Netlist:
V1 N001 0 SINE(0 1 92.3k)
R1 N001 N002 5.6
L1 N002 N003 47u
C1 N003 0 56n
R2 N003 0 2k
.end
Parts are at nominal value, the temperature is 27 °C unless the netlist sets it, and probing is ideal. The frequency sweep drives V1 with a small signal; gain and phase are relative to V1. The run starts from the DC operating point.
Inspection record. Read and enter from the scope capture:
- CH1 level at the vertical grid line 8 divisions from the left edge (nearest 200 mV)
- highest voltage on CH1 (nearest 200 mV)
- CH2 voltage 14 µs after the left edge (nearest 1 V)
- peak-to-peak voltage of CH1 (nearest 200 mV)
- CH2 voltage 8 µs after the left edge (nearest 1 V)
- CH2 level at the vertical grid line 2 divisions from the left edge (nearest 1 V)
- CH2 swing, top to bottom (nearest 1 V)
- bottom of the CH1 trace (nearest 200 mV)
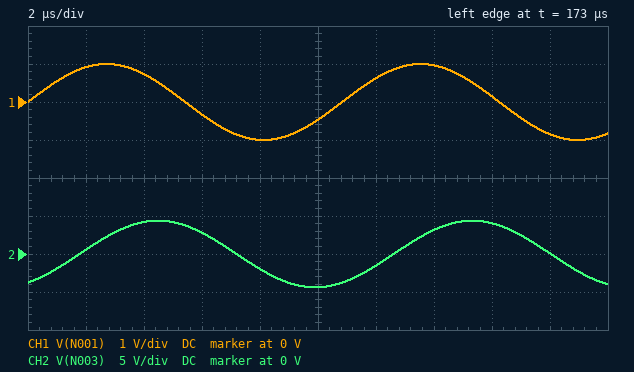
200 mV
1.0 V
3 V
2.0 V
-2 V
4 V
9 V
-1.0 V
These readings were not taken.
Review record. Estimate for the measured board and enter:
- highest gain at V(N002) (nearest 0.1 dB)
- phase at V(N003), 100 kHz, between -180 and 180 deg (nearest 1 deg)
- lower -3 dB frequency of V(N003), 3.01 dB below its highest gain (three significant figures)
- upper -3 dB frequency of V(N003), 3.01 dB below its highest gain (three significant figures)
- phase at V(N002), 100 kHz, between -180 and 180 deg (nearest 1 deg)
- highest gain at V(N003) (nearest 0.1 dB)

0 dB
-100 deg
86.3 kHz
107 kHz
60 deg
13.7 dB
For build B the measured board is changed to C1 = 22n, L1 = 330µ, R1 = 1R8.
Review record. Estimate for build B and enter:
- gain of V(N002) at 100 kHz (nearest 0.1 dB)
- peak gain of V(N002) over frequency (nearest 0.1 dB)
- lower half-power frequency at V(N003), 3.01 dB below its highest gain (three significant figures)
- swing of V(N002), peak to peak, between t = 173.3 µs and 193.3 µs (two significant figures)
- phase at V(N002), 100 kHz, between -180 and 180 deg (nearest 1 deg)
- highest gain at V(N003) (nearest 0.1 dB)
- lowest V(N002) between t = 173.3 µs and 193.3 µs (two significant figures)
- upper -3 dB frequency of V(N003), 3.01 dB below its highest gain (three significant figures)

0 dB
0 dB
56.7 kHz
2.0 V
1 deg
22.4 dB
-1.0 V
61.2 kHz
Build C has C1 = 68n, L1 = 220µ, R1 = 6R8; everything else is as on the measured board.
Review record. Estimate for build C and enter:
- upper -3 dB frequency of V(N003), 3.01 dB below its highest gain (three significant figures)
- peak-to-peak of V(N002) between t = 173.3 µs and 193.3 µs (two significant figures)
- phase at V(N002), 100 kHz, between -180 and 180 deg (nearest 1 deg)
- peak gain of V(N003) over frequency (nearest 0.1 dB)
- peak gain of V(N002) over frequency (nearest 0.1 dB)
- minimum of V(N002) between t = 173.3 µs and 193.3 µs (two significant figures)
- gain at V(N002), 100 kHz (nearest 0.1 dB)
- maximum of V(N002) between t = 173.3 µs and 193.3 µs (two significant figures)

43.9 kHz
2.0 V
3 deg
16.6 dB
0 dB
-1.0 V
0 dB
1.0 V
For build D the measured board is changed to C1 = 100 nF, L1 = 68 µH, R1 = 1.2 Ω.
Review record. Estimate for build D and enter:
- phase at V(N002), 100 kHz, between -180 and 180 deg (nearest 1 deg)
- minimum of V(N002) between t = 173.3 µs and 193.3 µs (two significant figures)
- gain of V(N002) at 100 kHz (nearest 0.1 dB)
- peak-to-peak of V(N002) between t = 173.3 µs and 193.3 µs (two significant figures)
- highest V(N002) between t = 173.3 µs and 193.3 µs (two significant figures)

3 deg
-1.0 V
0 dB
2.0 V
1.0 V
